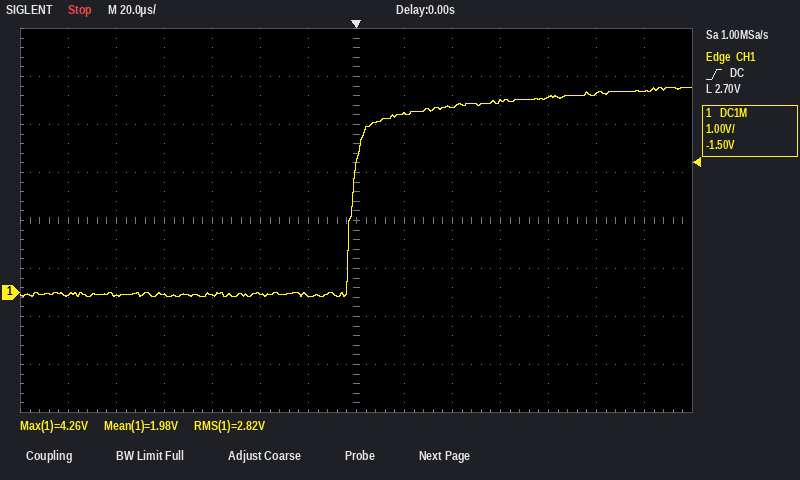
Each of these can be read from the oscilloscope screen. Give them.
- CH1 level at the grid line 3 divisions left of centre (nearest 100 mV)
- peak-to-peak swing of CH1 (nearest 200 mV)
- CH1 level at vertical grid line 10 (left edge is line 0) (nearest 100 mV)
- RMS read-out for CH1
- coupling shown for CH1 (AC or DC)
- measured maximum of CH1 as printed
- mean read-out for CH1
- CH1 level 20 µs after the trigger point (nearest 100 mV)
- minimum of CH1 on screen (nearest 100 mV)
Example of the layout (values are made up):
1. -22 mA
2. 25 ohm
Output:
1. -100 mV
2. 4.4 V
3. 4.0 V
4. 2.82 V
5. DC
6. 4.26 V
7. 1.98 V
8. 3.7 V
9. -100 mV
